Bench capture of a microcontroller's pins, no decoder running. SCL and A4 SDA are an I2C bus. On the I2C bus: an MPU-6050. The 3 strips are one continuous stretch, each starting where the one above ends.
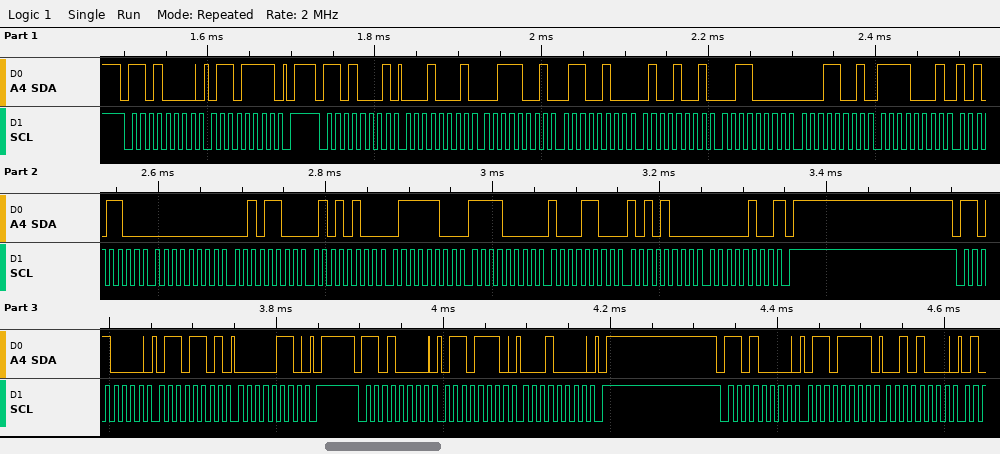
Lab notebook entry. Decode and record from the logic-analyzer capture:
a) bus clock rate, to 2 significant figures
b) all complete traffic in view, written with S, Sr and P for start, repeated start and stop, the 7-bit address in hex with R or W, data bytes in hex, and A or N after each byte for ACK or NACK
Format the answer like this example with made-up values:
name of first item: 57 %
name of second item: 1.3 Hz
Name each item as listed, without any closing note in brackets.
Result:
bus clock rate, to 2 significant figures: 100 kHz
all complete traffic in view, written with S, Sr and P for start, repeated start and stop, the 7-bit address in hex with R or W, data bytes in hex, and A or N after each byte for ACK or NACK: S 68W A 6F A P S 68R A 11 A 39 A 64 A 49 A 30 A 19 A F1 A AC A 00 A 2C A 54 A 7C A F0 A 8C A A8 A 04 N P S 68W A 6D A 06 A P S 68W A 6E A 10 A P S 68W A 6F A 28 A
